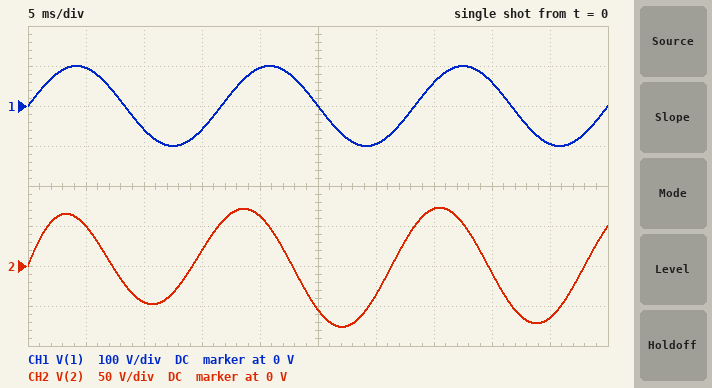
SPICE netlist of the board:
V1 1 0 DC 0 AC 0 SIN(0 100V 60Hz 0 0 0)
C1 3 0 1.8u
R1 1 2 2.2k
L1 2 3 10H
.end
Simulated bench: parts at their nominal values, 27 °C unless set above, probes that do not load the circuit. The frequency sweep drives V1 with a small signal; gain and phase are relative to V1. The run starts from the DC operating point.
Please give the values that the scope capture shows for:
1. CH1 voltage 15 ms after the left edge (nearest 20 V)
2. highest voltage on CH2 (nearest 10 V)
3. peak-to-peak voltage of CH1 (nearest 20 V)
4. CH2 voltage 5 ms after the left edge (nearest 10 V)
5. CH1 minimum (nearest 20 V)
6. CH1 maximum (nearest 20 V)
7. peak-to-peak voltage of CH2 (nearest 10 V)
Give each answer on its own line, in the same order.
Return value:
-60 V
70 V
200 V
50 V
-100 V
100 V
150 V
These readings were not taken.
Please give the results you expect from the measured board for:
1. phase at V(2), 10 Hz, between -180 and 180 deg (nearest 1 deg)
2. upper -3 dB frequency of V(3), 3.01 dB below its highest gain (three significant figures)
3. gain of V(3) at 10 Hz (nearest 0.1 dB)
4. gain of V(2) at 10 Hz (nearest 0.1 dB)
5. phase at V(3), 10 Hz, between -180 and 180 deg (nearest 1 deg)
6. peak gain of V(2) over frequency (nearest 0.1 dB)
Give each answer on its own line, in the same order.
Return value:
-15 deg
44.2 Hz
0.3 dB
-0.3 dB
-15 deg
0 dB
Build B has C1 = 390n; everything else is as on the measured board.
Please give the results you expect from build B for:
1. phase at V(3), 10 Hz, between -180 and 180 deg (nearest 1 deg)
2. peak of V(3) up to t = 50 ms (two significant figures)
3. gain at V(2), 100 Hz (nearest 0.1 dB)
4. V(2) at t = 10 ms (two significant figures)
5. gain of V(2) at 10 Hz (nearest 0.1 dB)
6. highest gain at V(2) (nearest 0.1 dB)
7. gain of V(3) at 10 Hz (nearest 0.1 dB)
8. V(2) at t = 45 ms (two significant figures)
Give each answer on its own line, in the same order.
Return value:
-3 deg
190 V
-3.0 dB
-8.4 V
0 dB
0 dB
0.1 dB
-48 V
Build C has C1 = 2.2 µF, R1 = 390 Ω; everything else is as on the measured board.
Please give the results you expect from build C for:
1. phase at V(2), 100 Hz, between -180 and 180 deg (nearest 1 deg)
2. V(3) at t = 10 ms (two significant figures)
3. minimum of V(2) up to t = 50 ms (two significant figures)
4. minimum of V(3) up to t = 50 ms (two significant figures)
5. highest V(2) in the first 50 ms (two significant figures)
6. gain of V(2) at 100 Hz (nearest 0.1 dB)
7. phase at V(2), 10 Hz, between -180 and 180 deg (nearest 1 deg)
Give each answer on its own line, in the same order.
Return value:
4 deg
87 V
-110 V
-100 V
100 V
0 dB
-3 deg
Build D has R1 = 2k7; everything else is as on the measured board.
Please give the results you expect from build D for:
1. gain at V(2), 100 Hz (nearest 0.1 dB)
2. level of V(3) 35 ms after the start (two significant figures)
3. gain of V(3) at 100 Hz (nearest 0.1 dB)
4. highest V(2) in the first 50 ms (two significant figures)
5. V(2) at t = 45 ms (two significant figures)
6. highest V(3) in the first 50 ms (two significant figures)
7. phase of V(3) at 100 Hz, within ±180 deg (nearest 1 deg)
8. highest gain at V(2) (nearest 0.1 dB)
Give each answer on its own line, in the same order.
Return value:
-1.0 dB
-41 V
-16.7 dB
66 V
-55 V
58 V
-153 deg
0 dB
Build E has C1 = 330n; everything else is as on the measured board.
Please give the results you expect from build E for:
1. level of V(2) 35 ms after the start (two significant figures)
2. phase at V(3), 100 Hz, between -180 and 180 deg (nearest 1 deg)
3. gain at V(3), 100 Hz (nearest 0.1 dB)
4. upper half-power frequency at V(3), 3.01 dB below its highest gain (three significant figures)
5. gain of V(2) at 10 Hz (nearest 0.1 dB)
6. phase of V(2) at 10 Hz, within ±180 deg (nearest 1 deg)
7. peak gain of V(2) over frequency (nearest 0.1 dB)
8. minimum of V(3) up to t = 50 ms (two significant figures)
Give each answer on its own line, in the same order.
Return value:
14 V
-124 deg
5.2 dB
100 Hz
0 dB
-3 deg
0 dB
-180 V
